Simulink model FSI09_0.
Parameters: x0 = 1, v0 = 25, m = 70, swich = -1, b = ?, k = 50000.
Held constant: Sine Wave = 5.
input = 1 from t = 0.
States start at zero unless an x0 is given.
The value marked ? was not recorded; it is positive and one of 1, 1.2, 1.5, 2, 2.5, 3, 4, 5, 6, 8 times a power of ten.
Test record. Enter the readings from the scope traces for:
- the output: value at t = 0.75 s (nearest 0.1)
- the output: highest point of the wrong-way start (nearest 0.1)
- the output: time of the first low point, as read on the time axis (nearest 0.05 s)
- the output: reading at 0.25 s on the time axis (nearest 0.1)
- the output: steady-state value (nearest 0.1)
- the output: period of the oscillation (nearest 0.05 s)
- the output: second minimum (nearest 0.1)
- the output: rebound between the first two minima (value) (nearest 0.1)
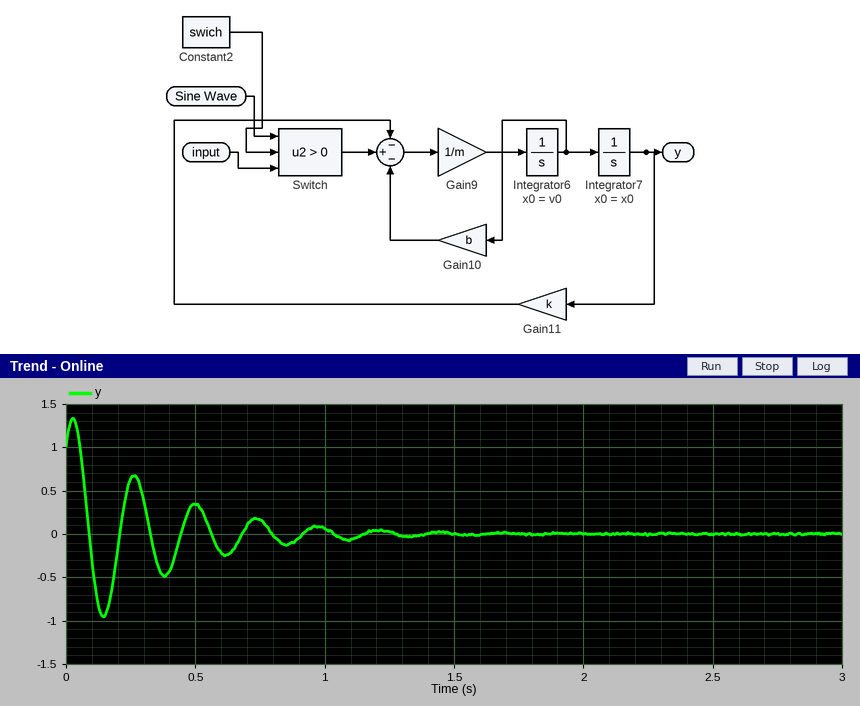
0.2
1.3
0.15 s
0.6
0.0
0.25 s
-0.5
0.7
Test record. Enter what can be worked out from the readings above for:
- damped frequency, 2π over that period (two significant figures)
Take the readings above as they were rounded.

25 rad/s
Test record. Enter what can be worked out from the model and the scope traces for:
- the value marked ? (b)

400
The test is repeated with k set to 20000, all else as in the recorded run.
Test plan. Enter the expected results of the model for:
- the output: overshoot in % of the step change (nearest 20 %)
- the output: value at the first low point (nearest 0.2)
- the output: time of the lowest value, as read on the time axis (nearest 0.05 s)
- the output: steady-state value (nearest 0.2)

100 %
-1.0
0.25 s
0.0
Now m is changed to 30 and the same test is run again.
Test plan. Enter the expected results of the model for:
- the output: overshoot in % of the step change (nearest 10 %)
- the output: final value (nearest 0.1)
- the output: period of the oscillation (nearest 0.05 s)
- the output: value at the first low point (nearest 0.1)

70 %
0.0
0.15 s
-0.7
